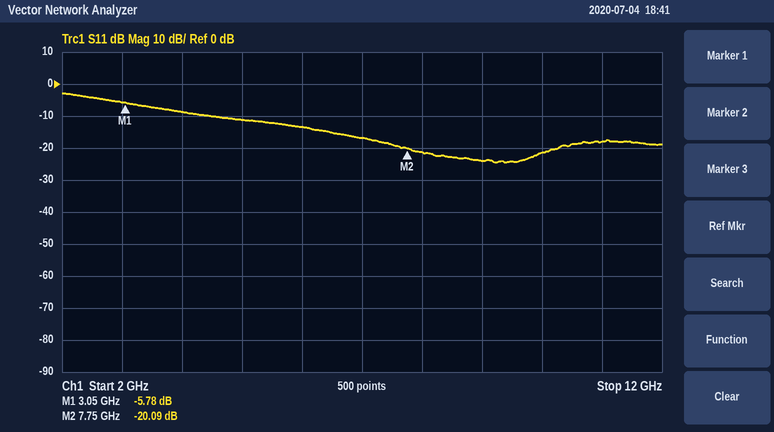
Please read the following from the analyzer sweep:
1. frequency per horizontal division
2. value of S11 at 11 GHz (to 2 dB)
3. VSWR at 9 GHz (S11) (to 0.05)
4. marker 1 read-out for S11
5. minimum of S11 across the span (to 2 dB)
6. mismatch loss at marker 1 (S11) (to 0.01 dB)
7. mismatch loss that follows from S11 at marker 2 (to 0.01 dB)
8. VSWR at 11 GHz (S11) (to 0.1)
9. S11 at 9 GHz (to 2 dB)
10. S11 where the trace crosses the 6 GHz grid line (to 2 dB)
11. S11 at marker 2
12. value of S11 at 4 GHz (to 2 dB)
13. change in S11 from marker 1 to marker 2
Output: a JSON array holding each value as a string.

["1 GHz", "-18 dB", "1.15", "-5.78 dB", "-24 dB", "1.33 dB", "0.04 dB", "1.3", "-24 dB", "-14 dB", "-20.09 dB", "-8 dB", "-14.31 dB"]
